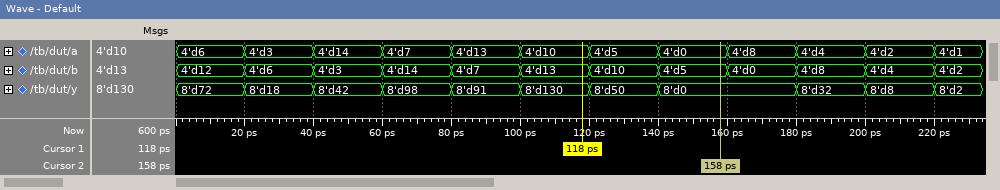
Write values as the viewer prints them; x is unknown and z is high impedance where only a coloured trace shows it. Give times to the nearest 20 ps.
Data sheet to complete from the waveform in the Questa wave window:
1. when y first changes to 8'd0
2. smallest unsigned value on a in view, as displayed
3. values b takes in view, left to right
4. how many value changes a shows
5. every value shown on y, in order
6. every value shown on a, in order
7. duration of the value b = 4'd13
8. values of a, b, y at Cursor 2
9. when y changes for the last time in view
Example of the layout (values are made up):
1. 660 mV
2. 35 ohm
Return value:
1. 140 ps
2. 4'd0
3. 4'd12, 4'd6, 4'd3, 4'd14, 4'd7, 4'd13, 4'd10, 4'd5, 4'd0, 4'd8, 4'd4, 4'd2
4. 11
5. 8'd72, 8'd18, 8'd42, 8'd98, 8'd91, 8'd130, 8'd50, 8'd0, 8'd32, 8'd8, 8'd2
6. 4'd6, 4'd3, 4'd14, 4'd7, 4'd13, 4'd10, 4'd5, 4'd0, 4'd8, 4'd4, 4'd2, 4'd1
7. 20 ps
8. a=4'd0, b=4'd5, y=8'd0
9. 220 ps
